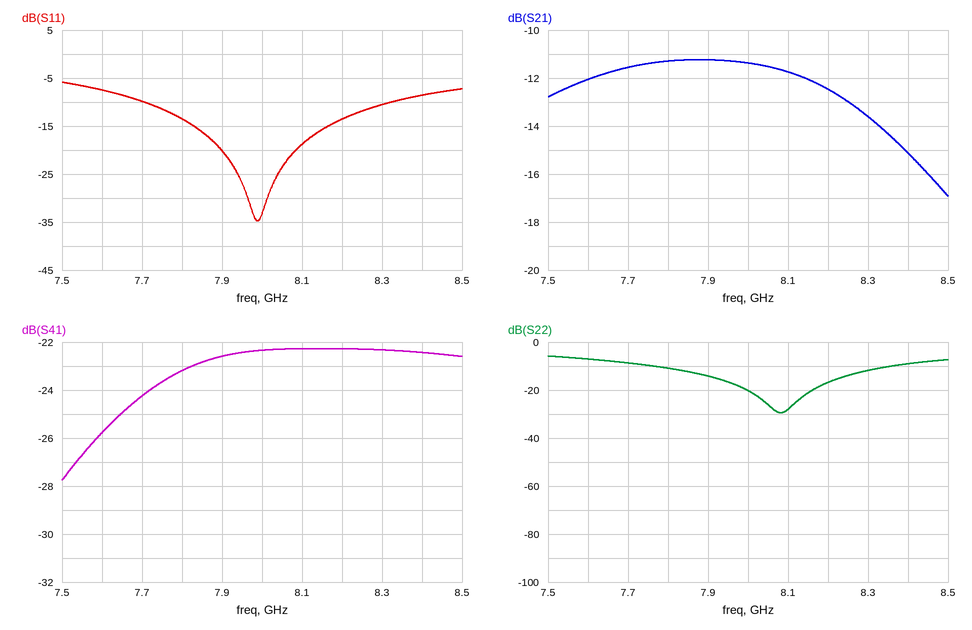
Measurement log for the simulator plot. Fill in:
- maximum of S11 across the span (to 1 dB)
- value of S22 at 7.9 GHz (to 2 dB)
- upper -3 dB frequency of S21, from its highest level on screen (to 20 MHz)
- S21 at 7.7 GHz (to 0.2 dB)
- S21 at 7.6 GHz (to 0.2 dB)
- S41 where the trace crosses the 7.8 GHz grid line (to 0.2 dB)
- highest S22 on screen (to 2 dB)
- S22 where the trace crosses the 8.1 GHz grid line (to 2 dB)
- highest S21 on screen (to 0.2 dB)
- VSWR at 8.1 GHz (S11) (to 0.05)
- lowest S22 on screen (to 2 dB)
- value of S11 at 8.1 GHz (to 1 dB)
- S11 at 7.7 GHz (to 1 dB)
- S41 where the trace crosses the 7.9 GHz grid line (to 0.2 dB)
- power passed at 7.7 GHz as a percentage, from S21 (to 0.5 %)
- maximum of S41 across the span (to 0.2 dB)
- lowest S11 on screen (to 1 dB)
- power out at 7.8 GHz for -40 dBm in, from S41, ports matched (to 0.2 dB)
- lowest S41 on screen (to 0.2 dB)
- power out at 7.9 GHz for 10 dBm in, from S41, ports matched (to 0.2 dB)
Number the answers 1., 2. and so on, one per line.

1. -6 dB
2. -14 dB
3. 8.34 GHz
4. -11.6 dB
5. -12.0 dB
6. -23.2 dB
7. -6 dB
8. -28 dB
9. -11.2 dB
10. 1.25
11. -30 dB
12. -19 dB
13. -10 dB
14. -22.6 dB
15. 7.0 %
16. -22.2 dB
17. -35 dB
18. -63.2 dBm
19. -27.8 dB
20. -12.6 dBm
